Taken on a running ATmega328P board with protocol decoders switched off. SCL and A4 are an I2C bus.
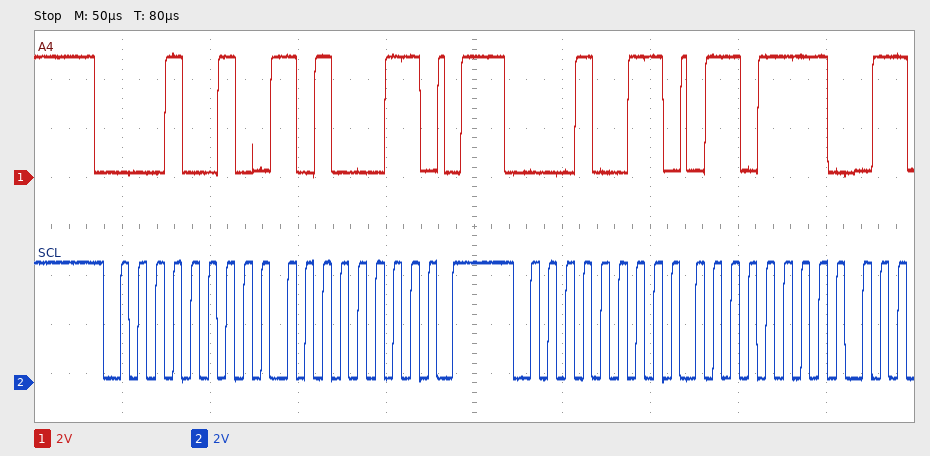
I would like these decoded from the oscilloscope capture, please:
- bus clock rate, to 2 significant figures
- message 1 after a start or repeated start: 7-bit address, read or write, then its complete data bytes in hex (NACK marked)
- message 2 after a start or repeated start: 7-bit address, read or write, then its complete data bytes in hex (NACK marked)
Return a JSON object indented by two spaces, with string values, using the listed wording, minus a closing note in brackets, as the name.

{
  "bus clock rate, to 2 significant figures": "100 kHz",
  "message 1 after a start or repeated start: 7-bit address, read or write, then its complete data bytes in hex": "0x09 write: A3",
  "message 2 after a start or repeated start: 7-bit address, read or write, then its complete data bytes in hex": "0x09 read: 6F"
}
